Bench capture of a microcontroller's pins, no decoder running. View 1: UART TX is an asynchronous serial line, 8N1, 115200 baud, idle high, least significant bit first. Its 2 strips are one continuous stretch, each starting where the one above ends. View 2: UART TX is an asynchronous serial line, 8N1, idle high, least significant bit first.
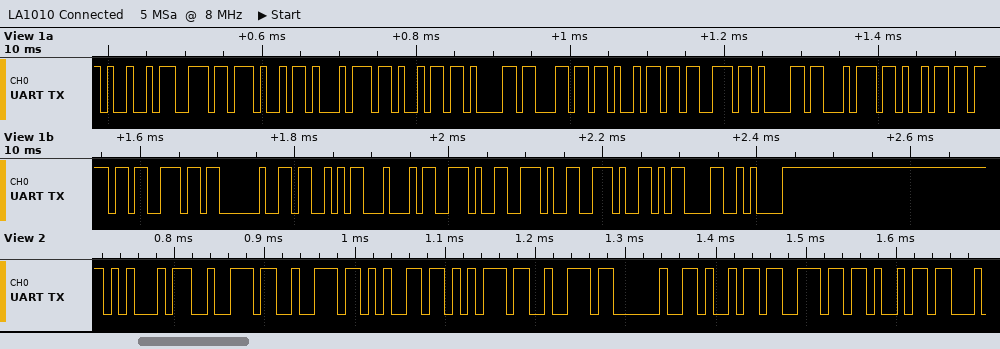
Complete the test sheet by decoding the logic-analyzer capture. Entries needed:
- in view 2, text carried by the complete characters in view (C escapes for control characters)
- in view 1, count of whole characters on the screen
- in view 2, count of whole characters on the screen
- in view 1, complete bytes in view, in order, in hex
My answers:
"Erreur ini"
22
10
49 6E 69 74 69 61 6C 69 73 61 74 69 6F 6E 20 53 44 2E 2E 2E 0D 0A
